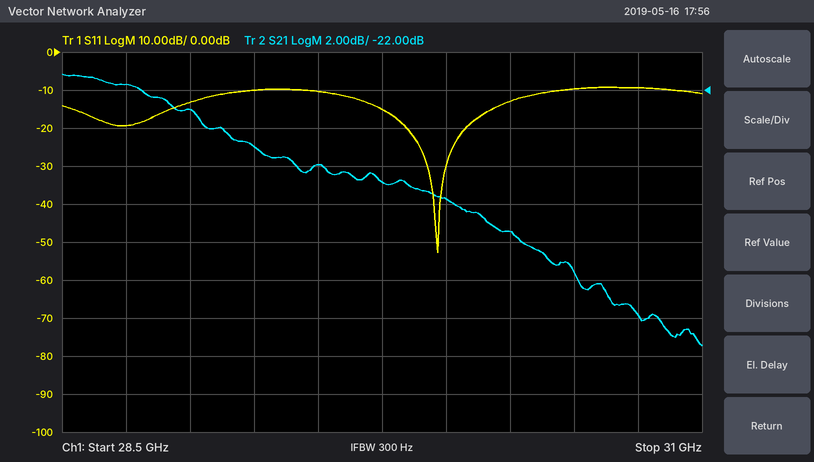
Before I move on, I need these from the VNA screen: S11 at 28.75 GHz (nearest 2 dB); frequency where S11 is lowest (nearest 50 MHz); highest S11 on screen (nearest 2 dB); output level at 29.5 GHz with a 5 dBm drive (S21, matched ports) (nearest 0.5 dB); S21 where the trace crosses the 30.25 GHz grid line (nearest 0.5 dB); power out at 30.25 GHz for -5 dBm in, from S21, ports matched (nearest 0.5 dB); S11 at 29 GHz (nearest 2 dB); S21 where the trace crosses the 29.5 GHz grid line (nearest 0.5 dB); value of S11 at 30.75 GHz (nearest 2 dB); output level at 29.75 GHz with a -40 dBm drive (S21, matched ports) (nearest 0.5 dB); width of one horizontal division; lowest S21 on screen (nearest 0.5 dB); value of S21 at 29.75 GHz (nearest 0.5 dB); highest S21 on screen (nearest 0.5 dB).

-20 dB
29.95 GHz
-10 dB
-21.0 dBm
-29.5 dB
-34.5 dBm
-14 dB
-26.0 dB
-10 dB
-67.0 dBm
250 MHz
-35.5 dB
-27.0 dB
-21.0 dB
